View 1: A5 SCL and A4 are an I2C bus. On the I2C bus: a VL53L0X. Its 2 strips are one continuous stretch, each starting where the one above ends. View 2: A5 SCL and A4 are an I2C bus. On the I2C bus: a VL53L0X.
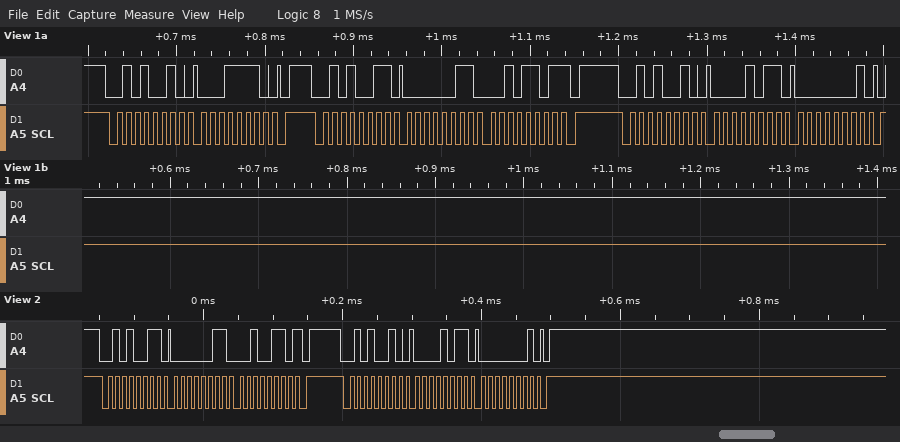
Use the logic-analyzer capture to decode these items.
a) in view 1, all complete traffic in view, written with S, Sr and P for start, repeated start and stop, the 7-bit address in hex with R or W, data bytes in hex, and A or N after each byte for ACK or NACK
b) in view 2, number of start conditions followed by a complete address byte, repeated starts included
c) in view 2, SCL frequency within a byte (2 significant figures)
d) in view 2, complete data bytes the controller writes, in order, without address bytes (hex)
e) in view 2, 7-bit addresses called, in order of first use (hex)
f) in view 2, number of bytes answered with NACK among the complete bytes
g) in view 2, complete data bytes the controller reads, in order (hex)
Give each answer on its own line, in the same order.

S 29W A 1E A P S 29R A 03 A 2D N P S 29W A 0B A 01 A P
2
100 kHz
0B 01
0x29
1
03 26
